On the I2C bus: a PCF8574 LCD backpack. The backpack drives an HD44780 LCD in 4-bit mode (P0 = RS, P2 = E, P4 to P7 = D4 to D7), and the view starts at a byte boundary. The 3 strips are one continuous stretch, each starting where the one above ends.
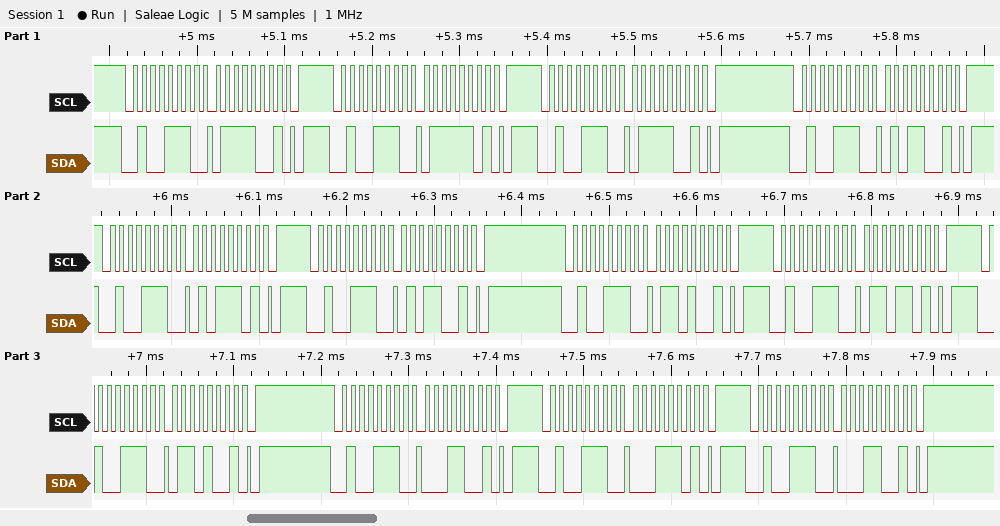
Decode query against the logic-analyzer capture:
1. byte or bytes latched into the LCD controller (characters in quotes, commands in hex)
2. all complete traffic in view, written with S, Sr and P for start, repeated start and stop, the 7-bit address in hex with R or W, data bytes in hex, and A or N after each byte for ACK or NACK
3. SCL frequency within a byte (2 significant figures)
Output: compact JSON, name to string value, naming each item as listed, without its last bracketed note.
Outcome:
{"byte or bytes latched into the LCD controller": "'u' 'a'", "all complete traffic in view, written with S, Sr and P for start, repeated start and stop, the 7-bit address in hex with R or W, data bytes in hex, and A or N after each byte for ACK or NACK": "S 27W A 79 A P S 27W A 7D A P S 27W A 79 A P S 27W A 59 A P S 27W A 5D A P S 27W A 59 A P S 27W A 69 A P S 27W A 6D A P S 27W A 69 A P S 27W A 19 A P S 27W A 1D A P S 27W A 19 A P", "SCL frequency within a byte": "100 kHz"}
